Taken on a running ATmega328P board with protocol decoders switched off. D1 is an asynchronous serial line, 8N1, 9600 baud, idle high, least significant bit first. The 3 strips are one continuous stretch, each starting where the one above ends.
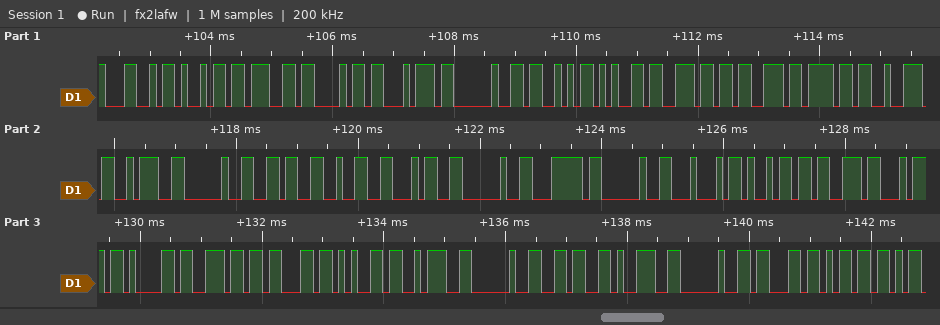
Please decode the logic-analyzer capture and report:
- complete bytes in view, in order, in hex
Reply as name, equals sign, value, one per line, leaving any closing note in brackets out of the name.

complete bytes in view, in order, in hex = 4C 69 67 68 74 20 53 65 6E 73 6F 72 3A 20 36 32 34 20 7C 20 44 69 73 74 61 6E 63 65 3A 20 36 39 20 63 6D
